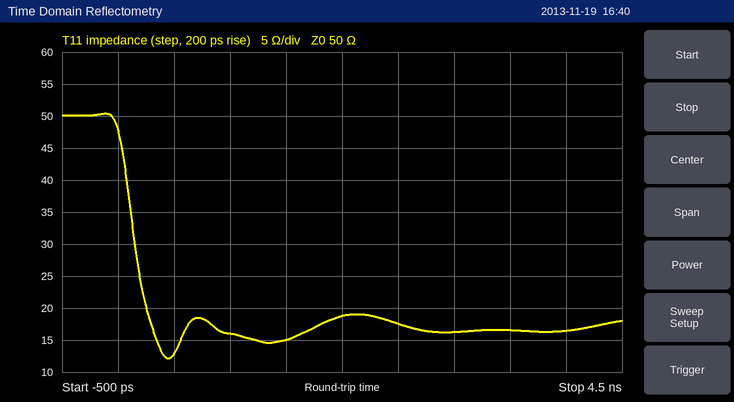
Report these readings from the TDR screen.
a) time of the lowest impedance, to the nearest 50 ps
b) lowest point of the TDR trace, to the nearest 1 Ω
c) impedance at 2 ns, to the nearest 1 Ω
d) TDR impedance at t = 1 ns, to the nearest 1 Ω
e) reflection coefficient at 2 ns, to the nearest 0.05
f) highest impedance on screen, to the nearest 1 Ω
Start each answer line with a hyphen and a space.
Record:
- 450 ps
- 12 Ω
- 19 Ω
- 16 Ω
- -0.45
- 50 Ω
